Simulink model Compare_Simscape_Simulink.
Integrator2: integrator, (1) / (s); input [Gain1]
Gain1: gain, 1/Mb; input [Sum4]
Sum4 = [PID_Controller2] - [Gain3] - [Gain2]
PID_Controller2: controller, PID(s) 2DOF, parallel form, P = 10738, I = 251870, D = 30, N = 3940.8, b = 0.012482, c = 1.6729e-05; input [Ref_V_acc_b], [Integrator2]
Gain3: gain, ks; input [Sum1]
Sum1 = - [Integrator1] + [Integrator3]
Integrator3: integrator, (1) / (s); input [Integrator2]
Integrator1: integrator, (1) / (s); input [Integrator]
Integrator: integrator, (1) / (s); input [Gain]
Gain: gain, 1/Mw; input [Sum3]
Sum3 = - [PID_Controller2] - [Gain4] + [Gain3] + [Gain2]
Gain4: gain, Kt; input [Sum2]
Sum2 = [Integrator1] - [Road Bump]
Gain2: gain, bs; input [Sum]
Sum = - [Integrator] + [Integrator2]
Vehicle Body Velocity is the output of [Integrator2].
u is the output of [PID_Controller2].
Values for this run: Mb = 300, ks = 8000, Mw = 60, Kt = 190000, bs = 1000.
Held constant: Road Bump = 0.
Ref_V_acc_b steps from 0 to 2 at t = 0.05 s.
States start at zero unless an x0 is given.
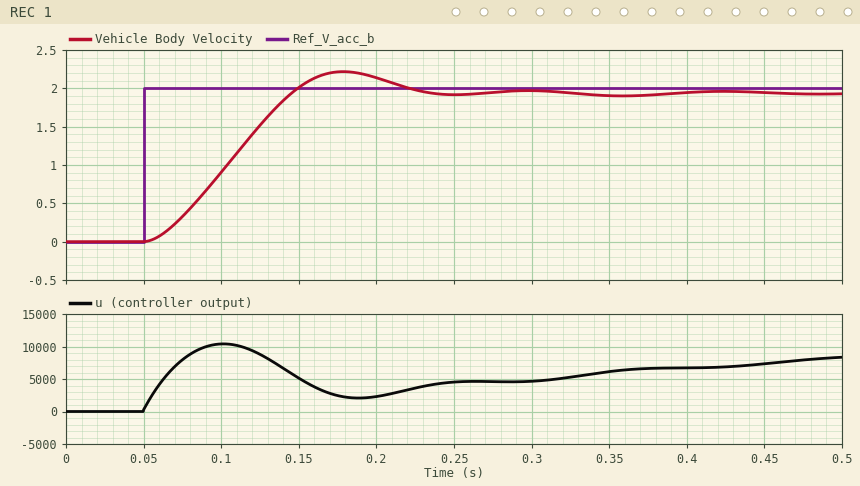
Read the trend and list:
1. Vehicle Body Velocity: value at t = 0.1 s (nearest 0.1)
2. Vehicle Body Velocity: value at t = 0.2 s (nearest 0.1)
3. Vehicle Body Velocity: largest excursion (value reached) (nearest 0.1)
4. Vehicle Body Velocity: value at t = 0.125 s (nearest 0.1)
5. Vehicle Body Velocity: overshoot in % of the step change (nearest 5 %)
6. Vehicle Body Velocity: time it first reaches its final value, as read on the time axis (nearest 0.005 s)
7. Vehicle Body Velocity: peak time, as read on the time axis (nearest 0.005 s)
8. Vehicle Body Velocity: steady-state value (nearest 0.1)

0.9
2.1
2.2
1.5
15 %
0.145 s
0.180 s
1.9
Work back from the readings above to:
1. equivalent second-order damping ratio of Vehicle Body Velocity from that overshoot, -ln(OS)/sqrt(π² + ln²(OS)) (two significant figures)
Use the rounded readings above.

0.52
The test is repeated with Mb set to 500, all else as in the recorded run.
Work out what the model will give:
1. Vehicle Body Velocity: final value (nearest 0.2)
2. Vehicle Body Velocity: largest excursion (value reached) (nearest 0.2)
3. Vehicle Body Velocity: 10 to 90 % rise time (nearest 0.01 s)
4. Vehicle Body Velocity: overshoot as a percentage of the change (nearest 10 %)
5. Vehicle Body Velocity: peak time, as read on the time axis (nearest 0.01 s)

2.0
2.4
0.07 s
20 %
0.20 s
